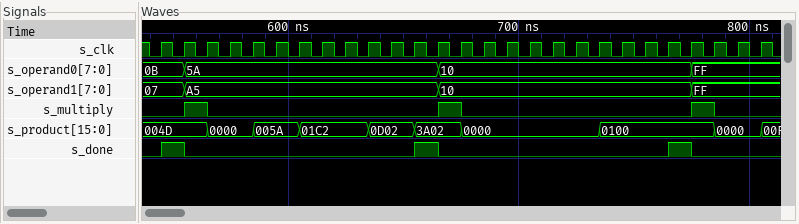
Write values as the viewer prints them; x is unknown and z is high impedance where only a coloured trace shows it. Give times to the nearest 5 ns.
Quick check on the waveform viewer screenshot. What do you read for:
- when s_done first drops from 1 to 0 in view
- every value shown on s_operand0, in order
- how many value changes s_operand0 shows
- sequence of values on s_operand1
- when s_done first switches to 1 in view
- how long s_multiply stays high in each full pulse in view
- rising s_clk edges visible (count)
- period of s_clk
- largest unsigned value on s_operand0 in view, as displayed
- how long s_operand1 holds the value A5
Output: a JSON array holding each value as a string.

["555 ns", "0B, 5A, 10, FF", "3", "07, A5, 10, FF", "545 ns", "10 ns, 10 ns, 10 ns", "27", "10 ns", "FF", "110 ns"]
